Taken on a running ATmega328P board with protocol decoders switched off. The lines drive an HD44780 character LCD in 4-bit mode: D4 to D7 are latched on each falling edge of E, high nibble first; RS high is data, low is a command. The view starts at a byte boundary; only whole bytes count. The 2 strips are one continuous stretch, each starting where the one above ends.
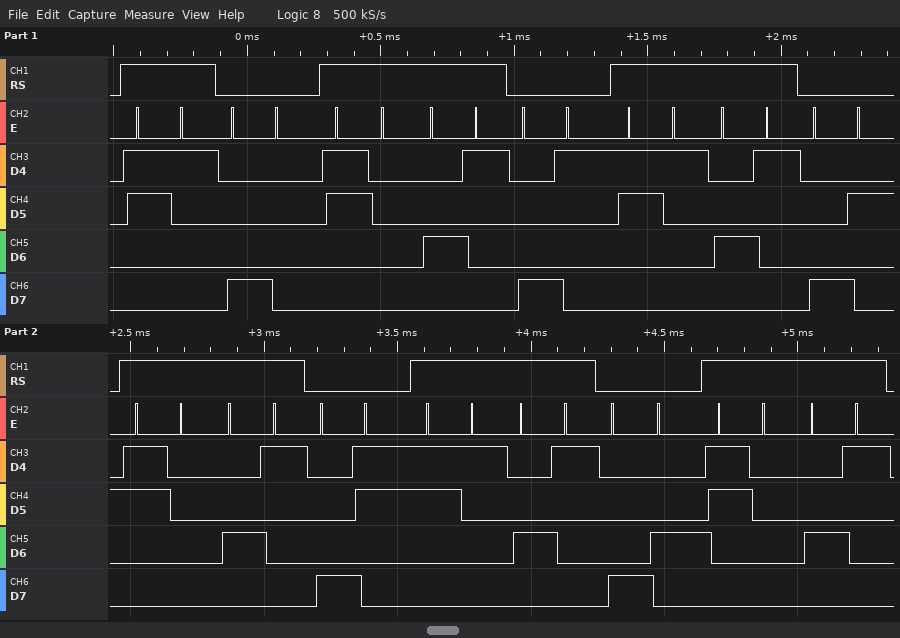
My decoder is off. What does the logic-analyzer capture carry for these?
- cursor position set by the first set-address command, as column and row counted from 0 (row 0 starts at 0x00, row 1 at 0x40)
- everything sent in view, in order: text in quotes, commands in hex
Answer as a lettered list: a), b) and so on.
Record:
a) column 0, row 0
b) "1" 0x80 "0A" 0x81 "1A" 0x82 "0A" 0x83 "1A" 0x84 "0A"
